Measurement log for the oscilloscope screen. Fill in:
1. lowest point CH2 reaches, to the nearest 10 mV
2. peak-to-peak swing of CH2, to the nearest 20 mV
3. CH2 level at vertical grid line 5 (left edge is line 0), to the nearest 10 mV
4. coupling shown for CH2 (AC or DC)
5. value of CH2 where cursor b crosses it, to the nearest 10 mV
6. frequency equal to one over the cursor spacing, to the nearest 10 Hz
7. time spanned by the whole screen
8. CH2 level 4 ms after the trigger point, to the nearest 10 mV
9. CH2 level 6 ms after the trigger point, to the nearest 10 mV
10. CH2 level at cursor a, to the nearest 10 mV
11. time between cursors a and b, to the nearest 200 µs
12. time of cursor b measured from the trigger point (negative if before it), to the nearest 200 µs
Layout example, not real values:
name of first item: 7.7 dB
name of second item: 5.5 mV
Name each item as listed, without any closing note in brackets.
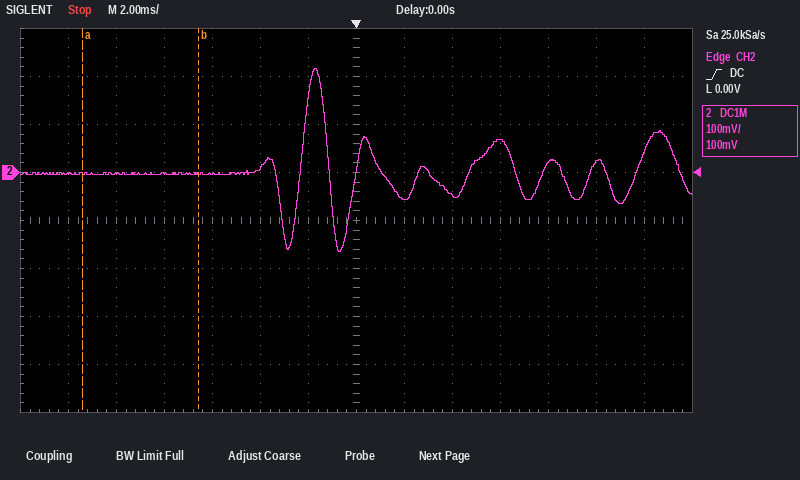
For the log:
lowest point CH2 reaches, to the nearest 10 mV: -160 mV
peak-to-peak swing of CH2, to the nearest 20 mV: 380 mV
CH2 level at vertical grid line 5 (left edge is line 0), to the nearest 10 mV: 10 mV
coupling shown for CH2: DC
value of CH2 where cursor b crosses it, to the nearest 10 mV: 0 mV
frequency equal to one over the cursor spacing, to the nearest 10 Hz: 210 Hz
time spanned by the whole screen: 28 ms
CH2 level 4 ms after the trigger point, to the nearest 10 mV: -50 mV
CH2 level 6 ms after the trigger point, to the nearest 10 mV: 70 mV
CH2 level at cursor a, to the nearest 10 mV: 0 mV
time between cursors a and b, to the nearest 200 µs: 4.8 ms
time of cursor b measured from the trigger point (negative if before it), to the nearest 200 µs: -6.6 ms
